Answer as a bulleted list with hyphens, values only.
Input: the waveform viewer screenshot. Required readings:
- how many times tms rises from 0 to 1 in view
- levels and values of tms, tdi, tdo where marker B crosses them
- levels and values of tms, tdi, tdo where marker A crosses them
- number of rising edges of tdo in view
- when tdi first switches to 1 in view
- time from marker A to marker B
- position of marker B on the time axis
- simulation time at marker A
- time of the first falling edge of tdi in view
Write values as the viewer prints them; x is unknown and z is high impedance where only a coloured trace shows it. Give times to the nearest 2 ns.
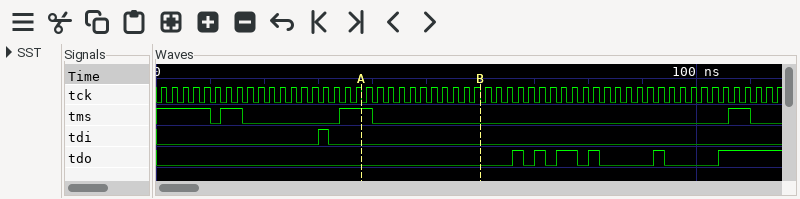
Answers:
- 3
- tms=0, tdi=0, tdo=0
- tms=1, tdi=0, tdo=0
- 6
- 30 ns
- 22 ns
- 60 ns
- 38 ns
- 32 ns
